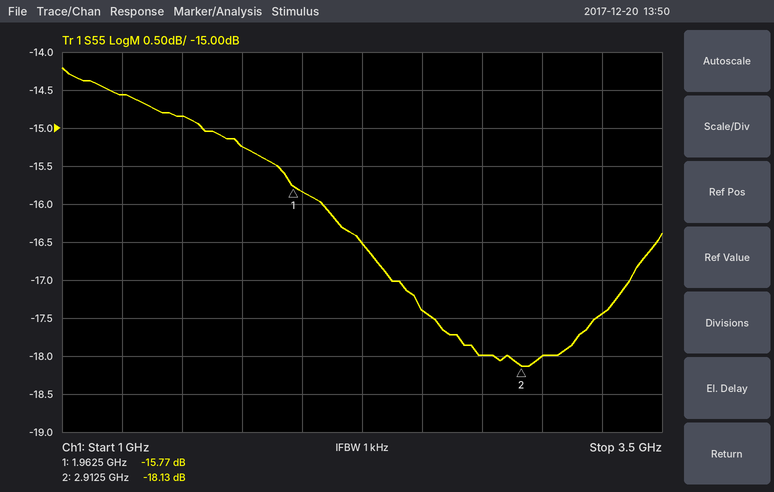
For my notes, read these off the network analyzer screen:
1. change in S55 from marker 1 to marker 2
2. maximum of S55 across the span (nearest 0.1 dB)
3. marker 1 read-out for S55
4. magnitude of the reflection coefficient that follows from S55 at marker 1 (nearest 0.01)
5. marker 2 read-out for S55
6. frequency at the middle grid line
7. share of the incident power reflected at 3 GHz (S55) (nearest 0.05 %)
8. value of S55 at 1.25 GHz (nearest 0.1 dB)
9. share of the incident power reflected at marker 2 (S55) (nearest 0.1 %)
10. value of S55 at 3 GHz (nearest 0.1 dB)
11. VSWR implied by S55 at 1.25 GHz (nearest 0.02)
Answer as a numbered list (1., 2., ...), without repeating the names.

1. -2.36 dB
2. -14.2 dB
3. -15.77 dB
4. 0.16
5. -18.13 dB
6. 2.25 GHz
7. 1.60 %
8. -14.6 dB
9. 1.5 %
10. -18.0 dB
11. 1.46
